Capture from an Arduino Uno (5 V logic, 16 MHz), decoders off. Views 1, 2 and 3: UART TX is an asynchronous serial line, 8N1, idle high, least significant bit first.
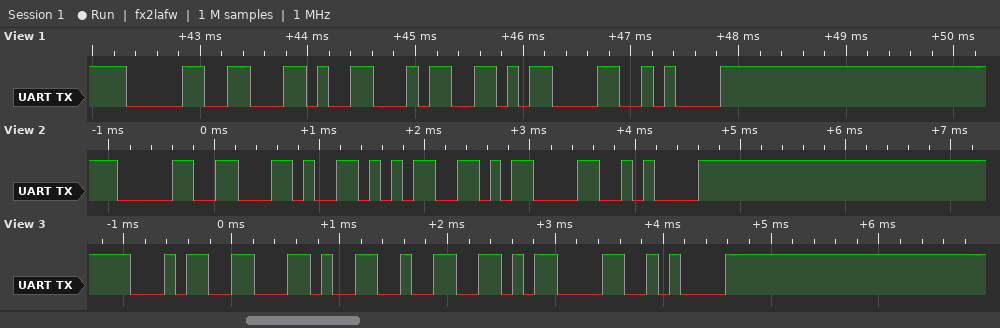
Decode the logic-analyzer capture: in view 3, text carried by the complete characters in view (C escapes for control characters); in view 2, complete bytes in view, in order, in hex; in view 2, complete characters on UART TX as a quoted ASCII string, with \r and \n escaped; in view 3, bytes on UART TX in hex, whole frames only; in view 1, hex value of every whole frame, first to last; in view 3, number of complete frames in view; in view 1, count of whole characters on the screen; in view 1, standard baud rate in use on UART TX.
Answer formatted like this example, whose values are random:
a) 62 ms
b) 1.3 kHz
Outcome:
a) "4,2\r\n"
b) 0x30 0x2C 0x35 0x0D 0x0A
c) "0,5\r\n"
d) 34 2C 32 0D 0A
e) 30 2C 34 0D 0A
f) 5
g) 5
h) 9600 baud
